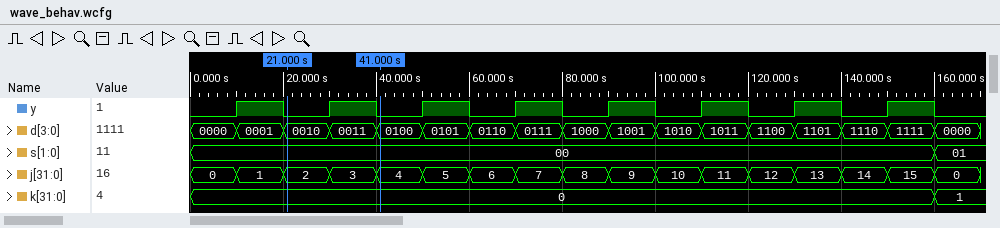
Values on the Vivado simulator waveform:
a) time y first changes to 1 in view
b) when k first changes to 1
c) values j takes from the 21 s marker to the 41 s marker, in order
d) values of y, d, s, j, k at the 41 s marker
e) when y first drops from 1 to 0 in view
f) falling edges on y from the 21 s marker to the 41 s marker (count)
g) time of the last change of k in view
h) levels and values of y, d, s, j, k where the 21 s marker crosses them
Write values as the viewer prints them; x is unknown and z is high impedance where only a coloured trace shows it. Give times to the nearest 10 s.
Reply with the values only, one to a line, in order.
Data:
10 s
160 s
2, 3, 4
y=0, d=0100, s=00, j=4, k=0
20 s
1
160 s
y=0, d=0010, s=00, j=2, k=0
